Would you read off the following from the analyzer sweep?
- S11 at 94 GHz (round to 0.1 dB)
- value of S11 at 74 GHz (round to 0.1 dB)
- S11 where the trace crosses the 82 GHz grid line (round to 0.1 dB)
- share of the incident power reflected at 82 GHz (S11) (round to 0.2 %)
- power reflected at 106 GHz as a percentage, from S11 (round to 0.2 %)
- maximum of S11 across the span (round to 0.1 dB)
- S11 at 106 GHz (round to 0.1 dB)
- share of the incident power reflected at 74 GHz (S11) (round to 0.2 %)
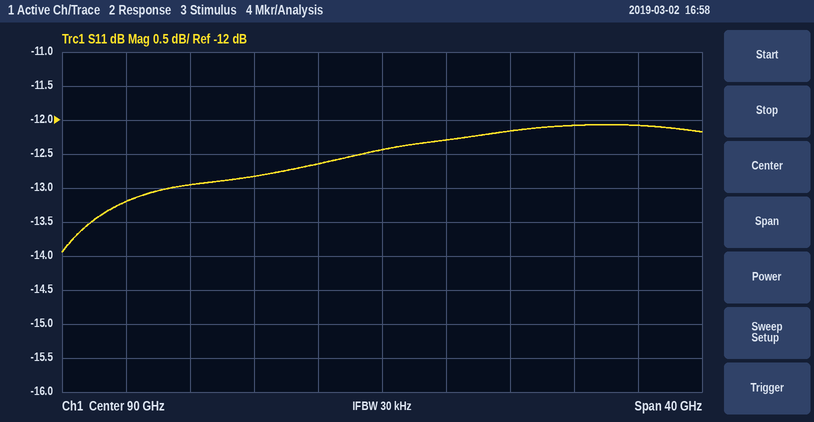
-12.3 dB
-13.2 dB
-12.8 dB
5.2 %
6.2 %
-12.1 dB
-12.1 dB
4.8 %
